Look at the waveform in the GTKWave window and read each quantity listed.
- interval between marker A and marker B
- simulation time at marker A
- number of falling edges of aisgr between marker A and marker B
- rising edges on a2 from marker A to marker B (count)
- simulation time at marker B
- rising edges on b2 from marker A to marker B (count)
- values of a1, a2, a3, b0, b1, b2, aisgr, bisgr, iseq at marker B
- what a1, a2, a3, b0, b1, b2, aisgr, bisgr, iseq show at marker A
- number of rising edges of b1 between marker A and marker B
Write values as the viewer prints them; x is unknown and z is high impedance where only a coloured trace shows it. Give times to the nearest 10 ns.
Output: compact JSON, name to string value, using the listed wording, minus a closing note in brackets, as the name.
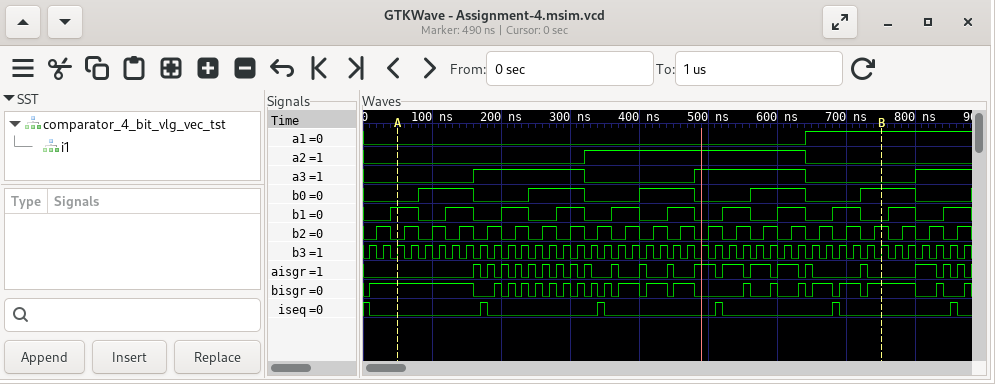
{"interval between marker A and marker B": "700 ns", "simulation time at marker A": "50 ns", "number of falling edges of aisgr between marker A and marker B": "18", "rising edges on a2 from marker A to marker B": "1", "simulation time at marker B": "750 ns", "rising edges on b2 from marker A to marker B": "18", "values of a1, a2, a3, b0, b1, b2, aisgr, bisgr, iseq at marker B": "a1=1, a2=0, a3=0, b0=1, b1=0, b2=1, aisgr=0, bisgr=1, iseq=0", "what a1, a2, a3, b0, b1, b2, aisgr, bisgr, iseq show at marker A": "a1=0, a2=0, a3=0, b0=0, b1=1, b2=0, aisgr=0, bisgr=1, iseq=0", "number of rising edges of b1 between marker A and marker B": "8"}
